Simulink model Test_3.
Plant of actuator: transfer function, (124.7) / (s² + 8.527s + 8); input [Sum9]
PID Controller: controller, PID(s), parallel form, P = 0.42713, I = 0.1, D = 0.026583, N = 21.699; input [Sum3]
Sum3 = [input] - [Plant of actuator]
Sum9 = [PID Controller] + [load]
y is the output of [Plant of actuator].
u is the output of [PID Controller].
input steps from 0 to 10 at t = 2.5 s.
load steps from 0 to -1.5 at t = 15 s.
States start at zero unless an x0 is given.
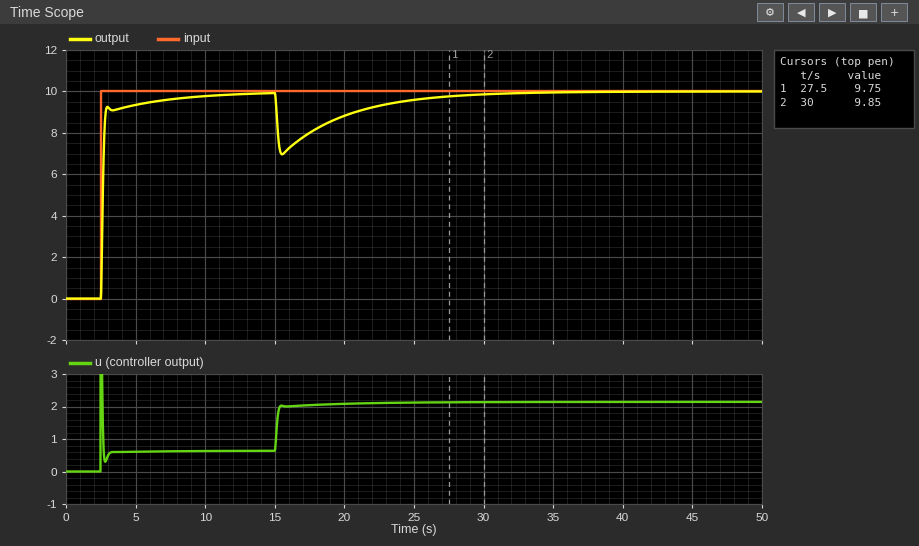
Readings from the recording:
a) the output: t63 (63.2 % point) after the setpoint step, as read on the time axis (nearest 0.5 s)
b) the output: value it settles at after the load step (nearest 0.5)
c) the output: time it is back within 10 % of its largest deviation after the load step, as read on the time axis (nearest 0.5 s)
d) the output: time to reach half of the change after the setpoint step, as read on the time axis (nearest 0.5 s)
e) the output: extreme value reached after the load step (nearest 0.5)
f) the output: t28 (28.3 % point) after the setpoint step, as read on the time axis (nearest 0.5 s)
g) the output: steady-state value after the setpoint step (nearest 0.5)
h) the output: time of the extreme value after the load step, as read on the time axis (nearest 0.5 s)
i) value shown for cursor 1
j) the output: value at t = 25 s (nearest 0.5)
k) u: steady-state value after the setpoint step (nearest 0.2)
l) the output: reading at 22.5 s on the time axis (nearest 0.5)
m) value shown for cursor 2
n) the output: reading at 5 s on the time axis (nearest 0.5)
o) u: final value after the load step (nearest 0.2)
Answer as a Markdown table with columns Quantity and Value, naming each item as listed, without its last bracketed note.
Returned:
| Quantity | Value |
|---|---|
| the output: t63 (63.2 % point) after the setpoint step, as read on the time axis | 2.5 s |
| the output: value it settles at after the load step | 10.0 |
| the output: time it is back within 10 % of its largest deviation after the load step, as read on the time axis | 26.5 s |
| the output: time to reach half of the change after the setpoint step, as read on the time axis | 2.5 s |
| the output: extreme value reached after the load step | 7.0 |
| the output: t28 (28.3 % point) after the setpoint step, as read on the time axis | 2.5 s |
| the output: steady-state value after the setpoint step | 10.0 |
| the output: time of the extreme value after the load step, as read on the time axis | 15.5 s |
| value shown for cursor 1 | 9.75 |
| the output: value at t = 25 s | 9.5 |
| u: steady-state value after the setpoint step | 0.6 |
| the output: reading at 22.5 s on the time axis | 9.5 |
| value shown for cursor 2 | 9.85 |
| the output: reading at 5 s on the time axis | 9.5 |
| u: final value after the load step | 2.2 |
